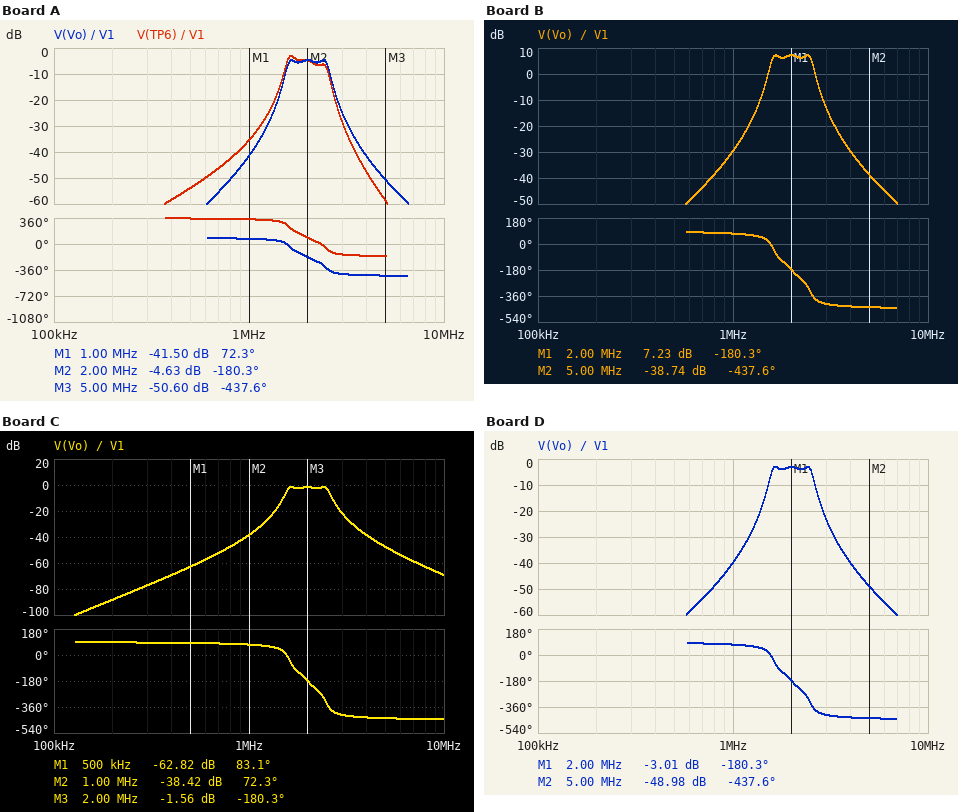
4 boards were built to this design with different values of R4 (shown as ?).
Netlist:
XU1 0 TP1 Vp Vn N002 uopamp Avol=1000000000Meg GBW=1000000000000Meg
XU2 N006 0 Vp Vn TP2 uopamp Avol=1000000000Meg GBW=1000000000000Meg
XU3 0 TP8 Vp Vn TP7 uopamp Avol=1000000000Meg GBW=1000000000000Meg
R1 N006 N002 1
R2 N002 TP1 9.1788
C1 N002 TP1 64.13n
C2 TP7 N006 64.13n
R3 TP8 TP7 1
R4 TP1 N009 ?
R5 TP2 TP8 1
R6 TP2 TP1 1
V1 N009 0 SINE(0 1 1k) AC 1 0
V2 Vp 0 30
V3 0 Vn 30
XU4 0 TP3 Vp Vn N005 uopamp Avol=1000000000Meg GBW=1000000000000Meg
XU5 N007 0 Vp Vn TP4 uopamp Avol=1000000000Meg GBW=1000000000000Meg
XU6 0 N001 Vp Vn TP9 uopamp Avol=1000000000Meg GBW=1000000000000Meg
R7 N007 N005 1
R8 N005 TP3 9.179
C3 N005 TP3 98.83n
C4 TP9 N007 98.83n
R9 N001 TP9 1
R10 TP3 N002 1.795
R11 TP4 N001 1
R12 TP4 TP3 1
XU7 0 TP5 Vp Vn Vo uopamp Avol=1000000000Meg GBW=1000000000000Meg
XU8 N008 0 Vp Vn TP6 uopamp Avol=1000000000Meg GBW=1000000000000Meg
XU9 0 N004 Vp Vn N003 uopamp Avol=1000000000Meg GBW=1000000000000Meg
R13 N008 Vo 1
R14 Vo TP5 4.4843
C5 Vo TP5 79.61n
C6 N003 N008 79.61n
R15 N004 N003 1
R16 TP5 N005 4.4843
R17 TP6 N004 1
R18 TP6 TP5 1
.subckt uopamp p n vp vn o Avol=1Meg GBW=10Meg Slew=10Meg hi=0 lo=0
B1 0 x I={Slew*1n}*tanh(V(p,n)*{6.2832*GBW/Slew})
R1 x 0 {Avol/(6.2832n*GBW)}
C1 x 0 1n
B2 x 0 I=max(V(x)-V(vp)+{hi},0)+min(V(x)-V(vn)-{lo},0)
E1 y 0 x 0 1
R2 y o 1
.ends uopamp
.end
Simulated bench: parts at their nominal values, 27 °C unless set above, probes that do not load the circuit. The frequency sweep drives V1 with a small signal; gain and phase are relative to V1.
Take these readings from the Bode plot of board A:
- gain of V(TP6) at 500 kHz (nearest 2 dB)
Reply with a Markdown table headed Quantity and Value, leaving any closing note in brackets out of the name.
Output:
| Quantity | Value |
|---|---|
| gain of V(TP6) at 500 kHz | -54 dB |
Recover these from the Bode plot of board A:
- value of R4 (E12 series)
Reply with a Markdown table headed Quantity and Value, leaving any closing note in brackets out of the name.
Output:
| Quantity | Value |
|---|---|
| value of R4 | 4.7 Ω |
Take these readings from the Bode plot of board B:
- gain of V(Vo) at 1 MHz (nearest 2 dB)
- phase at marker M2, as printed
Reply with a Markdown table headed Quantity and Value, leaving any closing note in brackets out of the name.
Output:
| Quantity | Value |
|---|---|
| gain of V(Vo) at 1 MHz | -30 dB |
| phase at marker M2, as printed | -437.6 deg |
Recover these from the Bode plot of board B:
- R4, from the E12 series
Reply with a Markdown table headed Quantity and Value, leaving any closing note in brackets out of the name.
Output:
| Quantity | Value |
|---|---|
| R4, from the E12 series | 1.2 Ω |
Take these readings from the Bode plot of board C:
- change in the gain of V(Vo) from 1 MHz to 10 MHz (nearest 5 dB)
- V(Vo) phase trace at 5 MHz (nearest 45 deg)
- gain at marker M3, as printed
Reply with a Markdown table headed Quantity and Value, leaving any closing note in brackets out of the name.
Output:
| Quantity | Value |
|---|---|
| change in the gain of V(Vo) from 1 MHz to 10 MHz | -30 dB |
| V(Vo) phase trace at 5 MHz | -450 deg |
| gain at marker M3, as printed | -1.56 dB |
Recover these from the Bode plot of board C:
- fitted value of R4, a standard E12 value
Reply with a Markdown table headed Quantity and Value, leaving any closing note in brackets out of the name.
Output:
| Quantity | Value |
|---|---|
| fitted value of R4, a standard E12 value | 3.3 Ω |
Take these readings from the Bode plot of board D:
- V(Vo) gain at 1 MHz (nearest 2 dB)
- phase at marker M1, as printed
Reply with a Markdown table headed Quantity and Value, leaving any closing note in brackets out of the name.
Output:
| Quantity | Value |
|---|---|
| V(Vo) gain at 1 MHz | -40 dB |
| phase at marker M1, as printed | -180.3 deg |
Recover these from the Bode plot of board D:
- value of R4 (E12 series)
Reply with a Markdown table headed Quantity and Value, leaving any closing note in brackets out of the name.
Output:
| Quantity | Value |
|---|---|
| value of R4 | 3.9 Ω |
